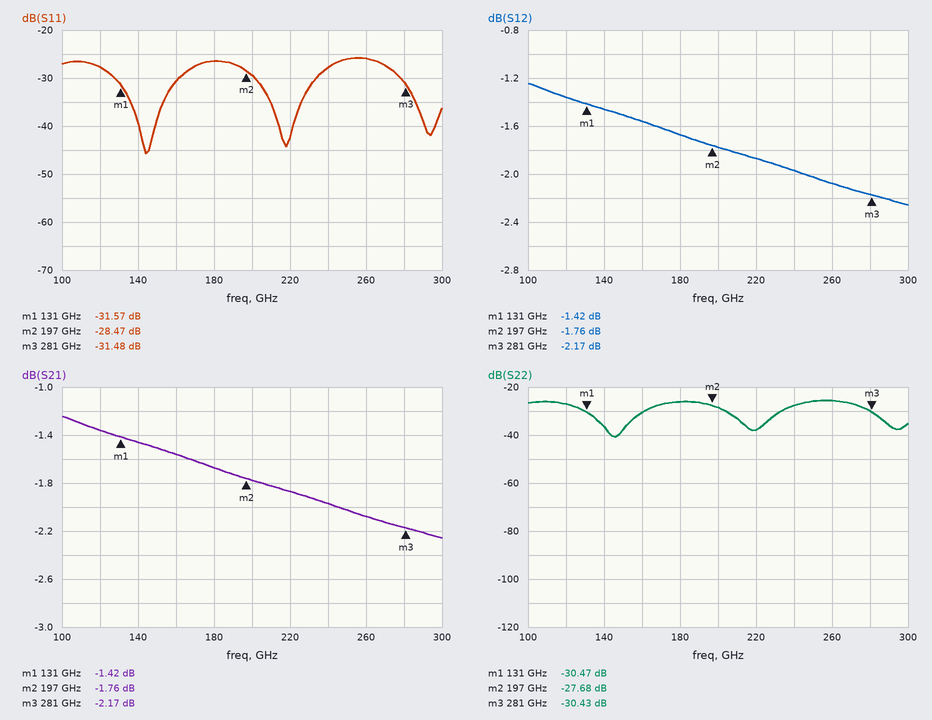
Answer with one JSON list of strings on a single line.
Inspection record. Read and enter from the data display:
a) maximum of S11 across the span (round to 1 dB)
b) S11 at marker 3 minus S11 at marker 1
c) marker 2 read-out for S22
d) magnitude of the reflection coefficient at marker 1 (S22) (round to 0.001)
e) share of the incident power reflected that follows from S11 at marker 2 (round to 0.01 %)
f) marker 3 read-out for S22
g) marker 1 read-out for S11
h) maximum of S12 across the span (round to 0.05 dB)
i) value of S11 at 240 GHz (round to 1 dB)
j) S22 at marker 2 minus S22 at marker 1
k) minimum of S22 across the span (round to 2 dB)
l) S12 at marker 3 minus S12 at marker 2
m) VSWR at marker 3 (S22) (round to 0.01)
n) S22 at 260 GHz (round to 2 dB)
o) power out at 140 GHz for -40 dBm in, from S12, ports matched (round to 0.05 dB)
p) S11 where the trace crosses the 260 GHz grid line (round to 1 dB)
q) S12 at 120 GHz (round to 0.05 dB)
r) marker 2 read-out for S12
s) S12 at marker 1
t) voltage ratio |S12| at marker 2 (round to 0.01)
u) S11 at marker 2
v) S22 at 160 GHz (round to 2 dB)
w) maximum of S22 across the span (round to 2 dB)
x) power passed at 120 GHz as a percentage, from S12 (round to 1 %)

["-26 dB", "0.09 dB", "-27.68 dB", "0.030", "0.14 %", "-30.43 dB", "-31.57 dB", "-1.25 dB", "-28 dB", "2.79 dB", "-40 dB", "-0.41 dB", "1.06", "-26 dB", "-41.45 dBm", "-26 dB", "-1.35 dB", "-1.76 dB", "-1.42 dB", "0.82", "-28.47 dB", "-30 dB", "-26 dB", "73 %"]
